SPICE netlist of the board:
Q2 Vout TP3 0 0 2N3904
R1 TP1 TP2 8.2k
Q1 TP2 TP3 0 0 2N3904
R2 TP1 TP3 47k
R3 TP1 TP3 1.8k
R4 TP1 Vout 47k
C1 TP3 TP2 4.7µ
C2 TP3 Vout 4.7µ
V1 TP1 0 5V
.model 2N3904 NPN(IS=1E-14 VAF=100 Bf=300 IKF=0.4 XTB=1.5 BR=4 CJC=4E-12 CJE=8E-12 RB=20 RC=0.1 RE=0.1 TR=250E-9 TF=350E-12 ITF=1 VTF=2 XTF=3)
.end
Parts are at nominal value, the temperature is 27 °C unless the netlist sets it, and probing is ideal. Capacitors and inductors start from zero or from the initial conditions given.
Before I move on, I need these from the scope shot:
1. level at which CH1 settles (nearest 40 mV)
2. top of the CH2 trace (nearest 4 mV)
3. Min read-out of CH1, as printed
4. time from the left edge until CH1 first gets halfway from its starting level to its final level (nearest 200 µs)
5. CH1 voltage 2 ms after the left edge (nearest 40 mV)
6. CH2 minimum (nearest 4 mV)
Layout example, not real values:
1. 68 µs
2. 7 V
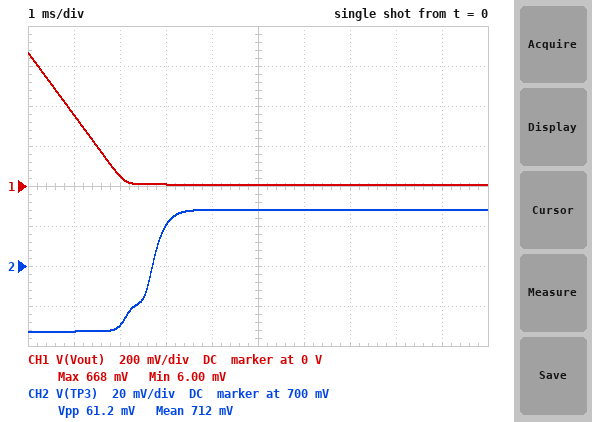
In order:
1. 0 V
2. 728 mV
3. 6.00 mV
4. 1.0 ms
5. 40 mV
6. 668 mV
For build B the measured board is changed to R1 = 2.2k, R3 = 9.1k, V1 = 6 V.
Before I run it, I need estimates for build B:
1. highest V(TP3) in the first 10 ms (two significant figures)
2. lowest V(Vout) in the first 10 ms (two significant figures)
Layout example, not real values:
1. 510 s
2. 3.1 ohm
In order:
1. 680 mV
2. 7.6 mV
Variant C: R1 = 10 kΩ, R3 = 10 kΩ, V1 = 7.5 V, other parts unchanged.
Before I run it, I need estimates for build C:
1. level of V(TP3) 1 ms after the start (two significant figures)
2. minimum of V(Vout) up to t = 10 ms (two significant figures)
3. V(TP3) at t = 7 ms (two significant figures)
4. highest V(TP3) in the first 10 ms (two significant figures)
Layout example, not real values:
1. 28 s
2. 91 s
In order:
1. 650 mV
2. 7.8 mV
3. 660 mV
4. 690 mV
